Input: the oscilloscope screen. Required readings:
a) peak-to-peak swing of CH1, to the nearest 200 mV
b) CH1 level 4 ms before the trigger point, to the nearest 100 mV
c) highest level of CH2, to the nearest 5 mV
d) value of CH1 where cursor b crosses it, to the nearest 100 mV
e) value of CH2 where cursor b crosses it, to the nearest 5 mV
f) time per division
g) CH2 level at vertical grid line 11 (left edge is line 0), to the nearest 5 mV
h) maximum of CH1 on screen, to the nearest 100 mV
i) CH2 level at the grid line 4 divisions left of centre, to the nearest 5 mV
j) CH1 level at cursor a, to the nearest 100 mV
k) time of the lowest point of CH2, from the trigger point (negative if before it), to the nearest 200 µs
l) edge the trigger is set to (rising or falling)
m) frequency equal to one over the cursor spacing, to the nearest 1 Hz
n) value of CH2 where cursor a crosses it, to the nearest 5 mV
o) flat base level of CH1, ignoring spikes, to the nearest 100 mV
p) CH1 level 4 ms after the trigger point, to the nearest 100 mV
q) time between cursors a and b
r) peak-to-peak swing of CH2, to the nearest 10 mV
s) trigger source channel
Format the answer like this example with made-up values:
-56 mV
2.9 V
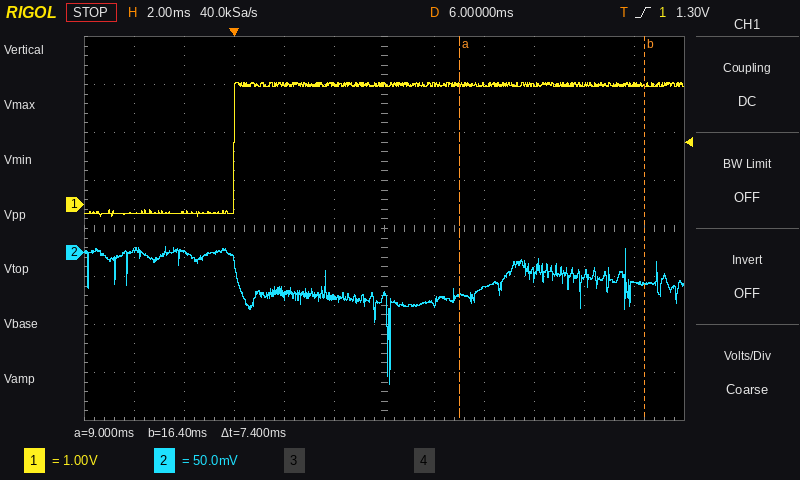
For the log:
2.8 V
-200 mV
5 mV
2.5 V
-35 mV
2 ms
-30 mV
2.5 V
0 mV
2.5 V
+6.2 ms
rising
135 Hz
-45 mV
-200 mV
2.5 V
7.4 ms
140 mV
CH1
